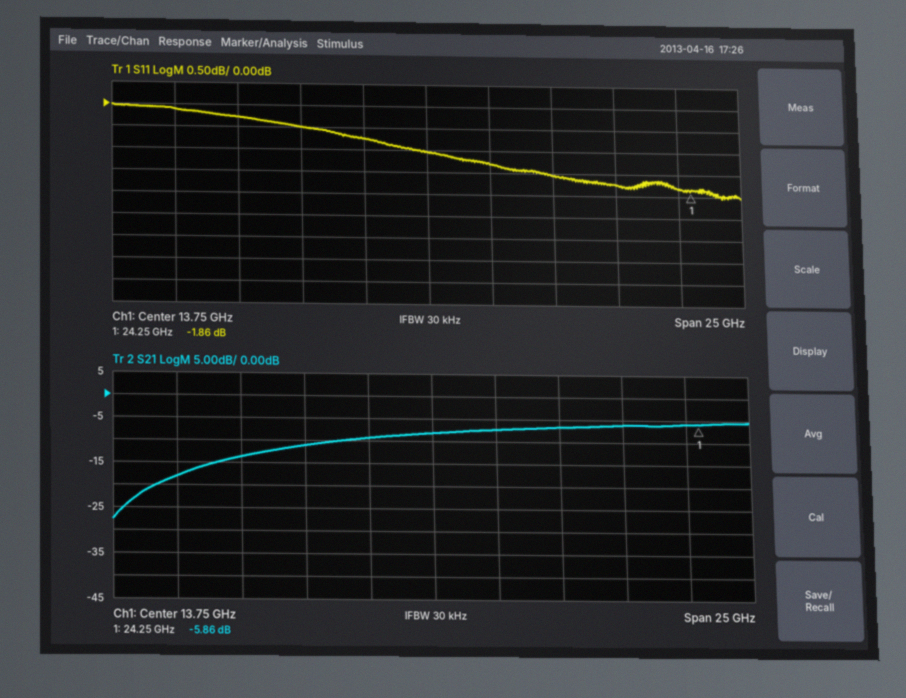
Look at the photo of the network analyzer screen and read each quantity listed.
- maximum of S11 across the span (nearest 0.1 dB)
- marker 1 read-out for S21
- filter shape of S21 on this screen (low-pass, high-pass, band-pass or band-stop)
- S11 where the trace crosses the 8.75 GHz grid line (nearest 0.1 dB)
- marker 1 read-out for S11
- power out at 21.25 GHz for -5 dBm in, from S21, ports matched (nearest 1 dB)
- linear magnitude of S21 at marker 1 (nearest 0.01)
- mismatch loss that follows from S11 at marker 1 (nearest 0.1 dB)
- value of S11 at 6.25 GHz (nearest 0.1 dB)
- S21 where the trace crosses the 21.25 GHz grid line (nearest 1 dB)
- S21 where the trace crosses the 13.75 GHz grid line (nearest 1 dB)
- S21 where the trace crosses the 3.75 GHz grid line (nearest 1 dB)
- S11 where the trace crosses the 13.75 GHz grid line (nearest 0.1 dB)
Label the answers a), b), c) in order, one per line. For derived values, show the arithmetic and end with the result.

a) 0.0 dB
b) -5.86 dB
c) high-pass
d) -0.5 dB
e) -1.86 dB
f) -5 dBm + (-6 dB) = -11 dBm
g) 10^(-5.86/20) ≈ 0.51
h) −10 log10(1 − 10^(-1.86/10)) ≈ 4.6 dB
i) -0.3 dB
j) -6 dB
k) -8 dB
l) -18 dB
m) -1.0 dB
